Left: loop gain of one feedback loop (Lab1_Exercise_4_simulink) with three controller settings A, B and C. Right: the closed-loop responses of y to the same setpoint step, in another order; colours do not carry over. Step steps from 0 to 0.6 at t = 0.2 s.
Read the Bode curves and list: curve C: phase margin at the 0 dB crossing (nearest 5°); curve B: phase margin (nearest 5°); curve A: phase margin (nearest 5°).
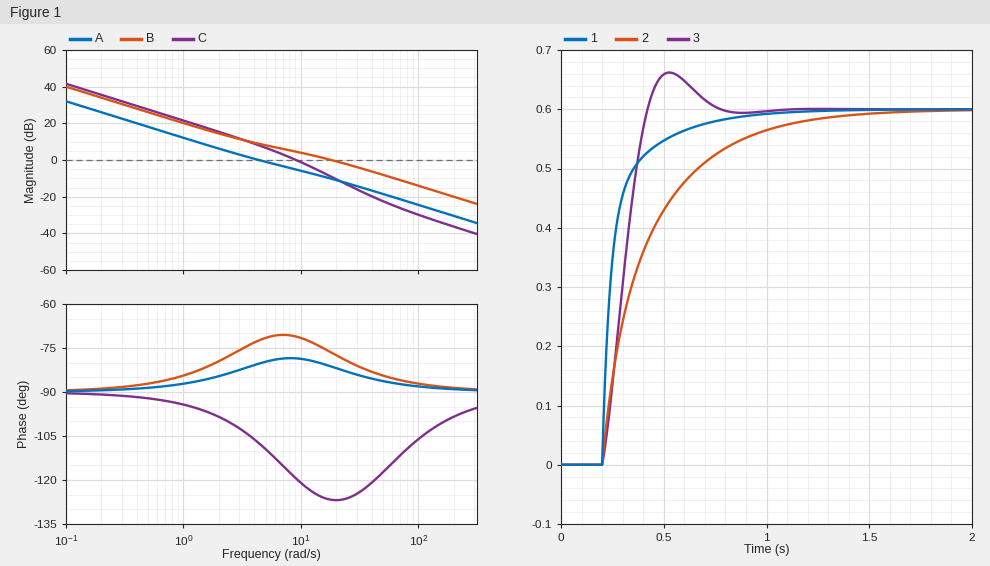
60°
105°
100°
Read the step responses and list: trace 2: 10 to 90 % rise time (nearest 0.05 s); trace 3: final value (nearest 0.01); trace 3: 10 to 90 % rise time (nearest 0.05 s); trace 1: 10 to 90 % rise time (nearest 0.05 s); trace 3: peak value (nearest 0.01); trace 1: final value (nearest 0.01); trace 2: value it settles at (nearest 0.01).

0.60 s
0.60
0.15 s
0.25 s
0.66
0.60
0.60
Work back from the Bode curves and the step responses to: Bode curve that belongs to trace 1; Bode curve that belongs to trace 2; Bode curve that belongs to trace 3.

B
A
C
